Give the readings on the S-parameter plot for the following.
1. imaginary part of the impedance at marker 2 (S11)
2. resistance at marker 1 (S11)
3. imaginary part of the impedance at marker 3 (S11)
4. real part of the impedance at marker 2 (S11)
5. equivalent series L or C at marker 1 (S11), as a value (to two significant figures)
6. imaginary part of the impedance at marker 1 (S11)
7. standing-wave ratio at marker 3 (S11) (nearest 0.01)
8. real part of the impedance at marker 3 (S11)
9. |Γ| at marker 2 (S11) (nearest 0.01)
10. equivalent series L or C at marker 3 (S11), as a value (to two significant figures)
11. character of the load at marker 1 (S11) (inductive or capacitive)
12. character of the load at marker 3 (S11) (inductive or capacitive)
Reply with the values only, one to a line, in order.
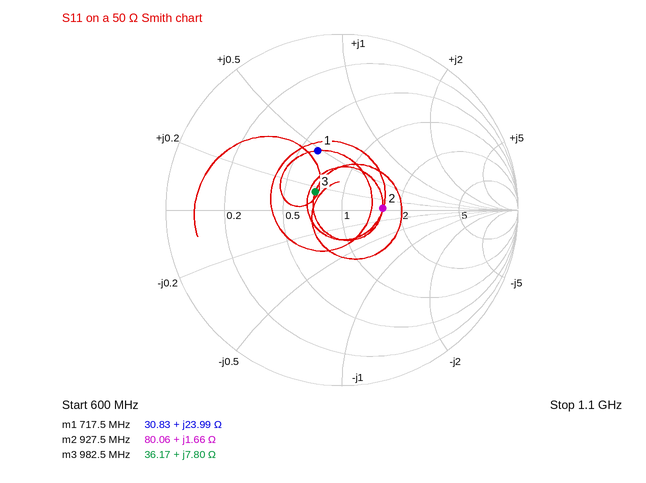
+1.66 Ω
30.83 Ω
+7.80 Ω
80.06 Ω
5.3 nH
+23.99 Ω
1.45
36.17 Ω
0.23
1.3 nH
inductive
inductive
